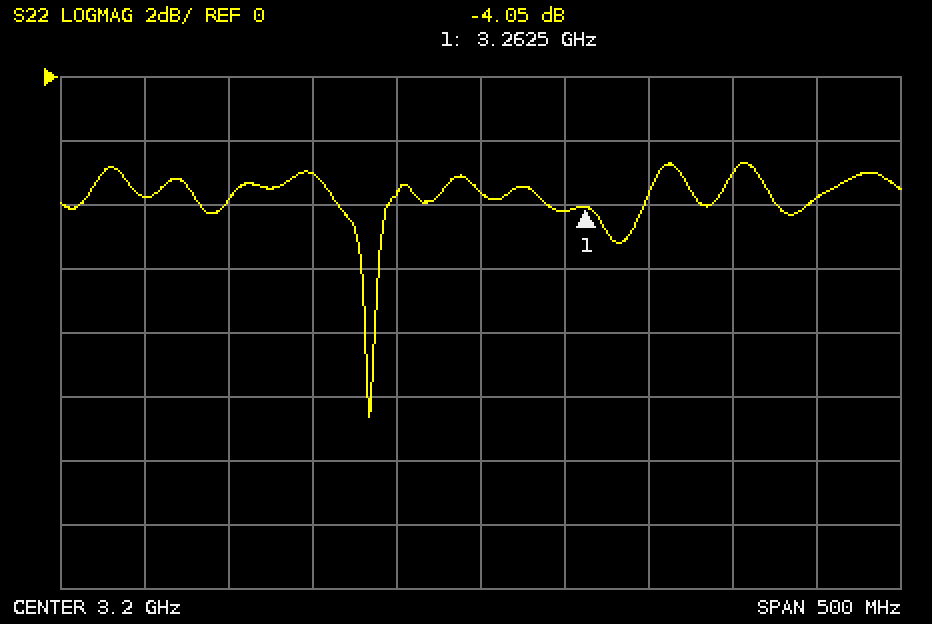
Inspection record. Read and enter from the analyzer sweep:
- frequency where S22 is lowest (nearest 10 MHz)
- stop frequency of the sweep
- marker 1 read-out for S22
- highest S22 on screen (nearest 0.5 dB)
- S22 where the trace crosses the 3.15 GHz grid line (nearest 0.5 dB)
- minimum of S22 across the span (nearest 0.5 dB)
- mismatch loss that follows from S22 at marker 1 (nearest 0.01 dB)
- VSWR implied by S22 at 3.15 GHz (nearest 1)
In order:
3.13 GHz
3.45 GHz
-4.05 dB
-2.5 dB
-3.5 dB
-10.5 dB
2.17 dB
5
